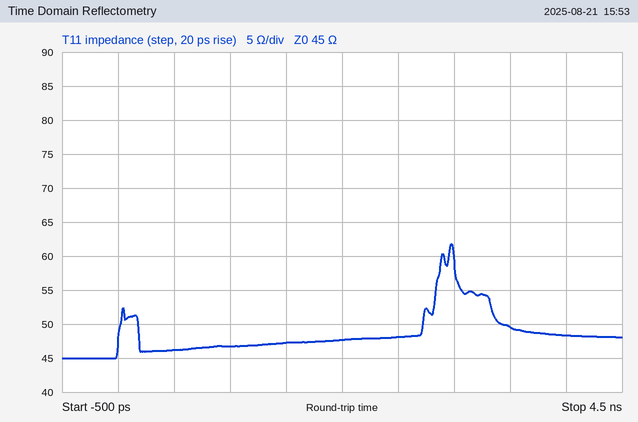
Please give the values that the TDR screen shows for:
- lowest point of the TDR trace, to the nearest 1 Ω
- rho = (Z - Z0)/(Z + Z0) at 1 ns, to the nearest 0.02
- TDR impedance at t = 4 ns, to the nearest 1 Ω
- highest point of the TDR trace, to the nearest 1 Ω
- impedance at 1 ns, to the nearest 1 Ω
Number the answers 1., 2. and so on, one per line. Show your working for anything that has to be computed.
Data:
1. 45 Ω
2. (47 − 45)/(47 + 45) ≈ +0.02
3. 48 Ω
4. 62 Ω
5. 47 Ω
